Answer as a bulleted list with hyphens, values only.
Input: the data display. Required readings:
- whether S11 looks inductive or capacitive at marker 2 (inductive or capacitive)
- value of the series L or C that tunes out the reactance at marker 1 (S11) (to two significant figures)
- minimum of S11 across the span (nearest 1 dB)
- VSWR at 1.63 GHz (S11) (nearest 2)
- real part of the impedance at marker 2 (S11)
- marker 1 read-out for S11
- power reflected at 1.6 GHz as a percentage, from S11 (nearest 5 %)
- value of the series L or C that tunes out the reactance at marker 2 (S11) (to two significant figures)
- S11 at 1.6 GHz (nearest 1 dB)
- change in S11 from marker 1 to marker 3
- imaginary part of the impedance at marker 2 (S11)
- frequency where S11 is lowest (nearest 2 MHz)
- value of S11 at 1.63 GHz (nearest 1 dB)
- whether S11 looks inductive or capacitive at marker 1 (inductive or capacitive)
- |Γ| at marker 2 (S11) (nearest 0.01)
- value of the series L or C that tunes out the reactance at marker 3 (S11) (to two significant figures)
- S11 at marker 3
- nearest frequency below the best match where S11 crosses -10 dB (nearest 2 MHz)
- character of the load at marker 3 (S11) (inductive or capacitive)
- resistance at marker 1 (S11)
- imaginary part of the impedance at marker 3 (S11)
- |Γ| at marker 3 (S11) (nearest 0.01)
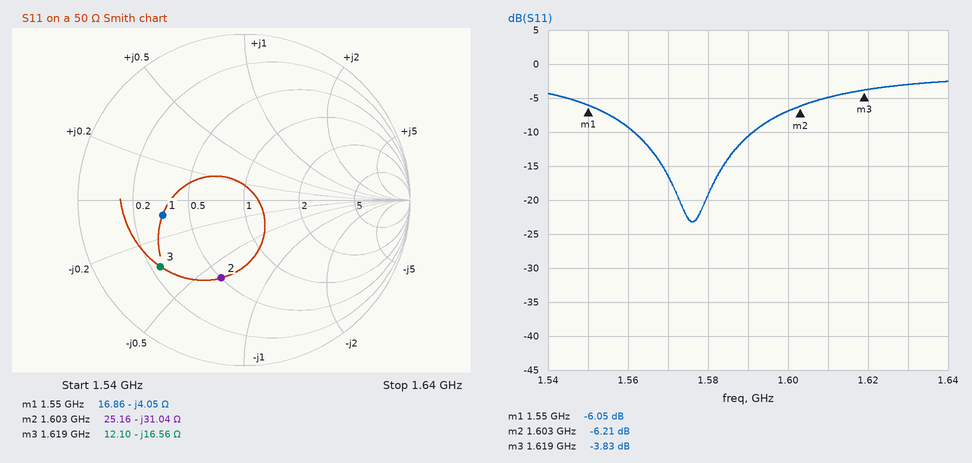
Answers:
- capacitive
- 420 pH
- -23 dB
- 6
- 25.16 Ω
- -6.05 dB
- 20 %
- 3.1 nH
- -7 dB
- 2.22 dB
- -31.04 Ω
- 1.576 GHz
- -3 dB
- capacitive
- 0.49
- 1.6 nH
- -3.83 dB
- 1.562 GHz
- capacitive
- 16.86 Ω
- -16.56 Ω
- 0.64
